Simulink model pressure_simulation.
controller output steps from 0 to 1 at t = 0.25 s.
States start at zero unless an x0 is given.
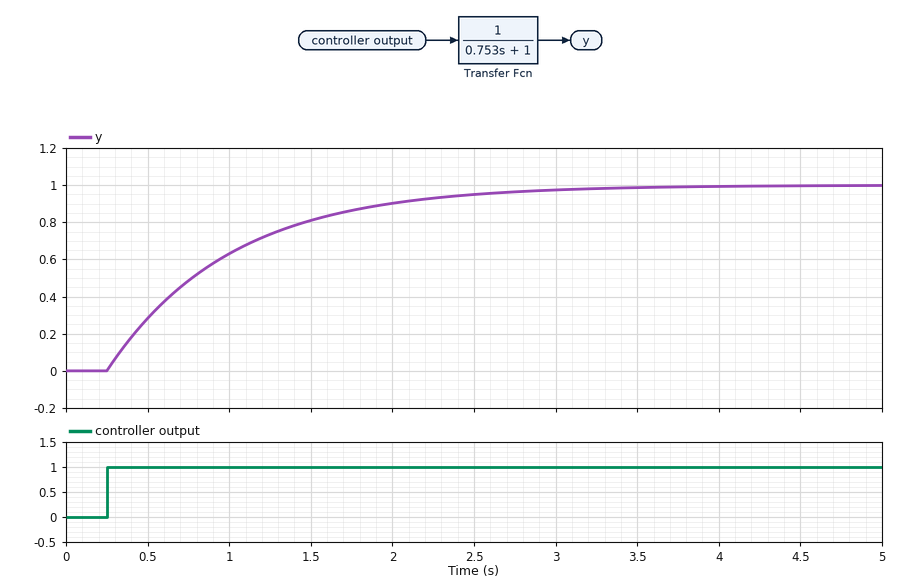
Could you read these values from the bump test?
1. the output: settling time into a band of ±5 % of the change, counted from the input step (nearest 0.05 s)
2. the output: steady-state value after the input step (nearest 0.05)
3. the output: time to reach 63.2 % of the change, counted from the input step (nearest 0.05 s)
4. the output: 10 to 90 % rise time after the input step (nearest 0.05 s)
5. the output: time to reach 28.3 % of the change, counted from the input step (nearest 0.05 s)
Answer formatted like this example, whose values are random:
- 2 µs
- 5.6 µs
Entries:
- 2.25 s
- 1.00
- 0.75 s
- 1.65 s
- 0.25 s
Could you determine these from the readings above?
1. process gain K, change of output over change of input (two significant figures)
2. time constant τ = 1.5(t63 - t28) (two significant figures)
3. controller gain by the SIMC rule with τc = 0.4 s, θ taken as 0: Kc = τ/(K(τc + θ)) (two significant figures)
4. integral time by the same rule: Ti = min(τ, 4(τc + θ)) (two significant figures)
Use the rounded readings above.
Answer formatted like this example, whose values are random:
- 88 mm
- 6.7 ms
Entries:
- 1.0
- 0.75 s
- 1.9
- 0.75 s
